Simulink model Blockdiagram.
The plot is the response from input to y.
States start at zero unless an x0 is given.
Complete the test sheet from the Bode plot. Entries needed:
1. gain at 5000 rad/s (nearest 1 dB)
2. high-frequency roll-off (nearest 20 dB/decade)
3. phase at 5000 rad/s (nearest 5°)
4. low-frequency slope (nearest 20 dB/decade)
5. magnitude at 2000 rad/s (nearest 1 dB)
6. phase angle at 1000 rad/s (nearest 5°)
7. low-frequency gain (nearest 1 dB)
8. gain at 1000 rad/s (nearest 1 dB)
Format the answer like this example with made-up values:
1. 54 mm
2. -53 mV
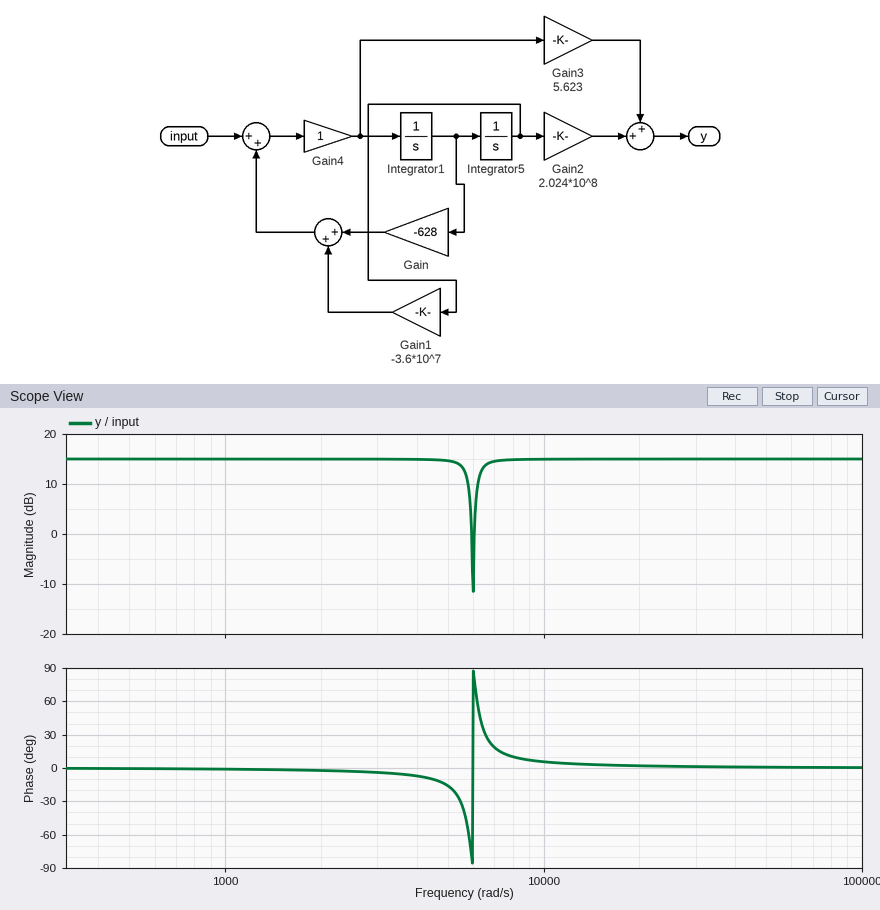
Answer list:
1. 15 dB
2. 0 dB/decade
3. -15°
4. 0 dB/decade
5. 15 dB
6. 0°
7. 15 dB
8. 15 dB
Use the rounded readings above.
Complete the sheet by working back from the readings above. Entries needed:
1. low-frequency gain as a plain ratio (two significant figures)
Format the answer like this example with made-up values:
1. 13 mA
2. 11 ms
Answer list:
1. 5.6
